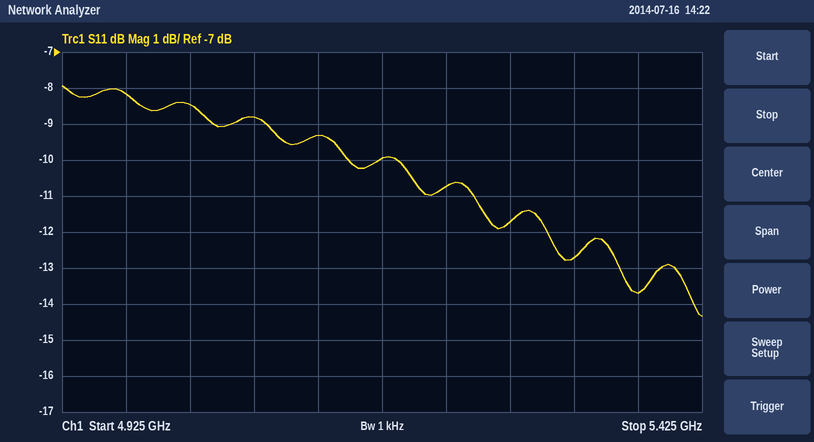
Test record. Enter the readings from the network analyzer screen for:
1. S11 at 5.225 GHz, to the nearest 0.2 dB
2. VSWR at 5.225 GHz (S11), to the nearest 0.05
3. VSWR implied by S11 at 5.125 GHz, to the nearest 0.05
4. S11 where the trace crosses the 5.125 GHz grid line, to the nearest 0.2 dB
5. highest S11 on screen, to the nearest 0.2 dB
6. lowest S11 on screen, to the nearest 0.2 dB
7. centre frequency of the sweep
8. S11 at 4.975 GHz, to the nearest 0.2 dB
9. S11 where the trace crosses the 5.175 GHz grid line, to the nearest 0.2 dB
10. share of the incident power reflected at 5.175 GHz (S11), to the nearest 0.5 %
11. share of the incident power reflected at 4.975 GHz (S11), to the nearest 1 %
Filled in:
-10.8 dB
1.80
2.05
-9.4 dB
-8.0 dB
-14.4 dB
5.175 GHz
-8.2 dB
-10.0 dB
10.0 %
15 %
